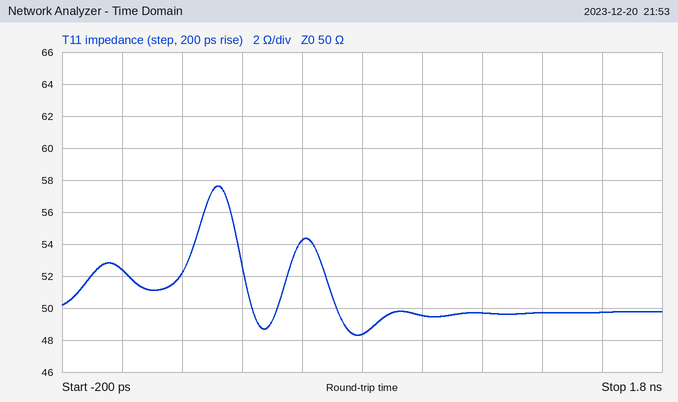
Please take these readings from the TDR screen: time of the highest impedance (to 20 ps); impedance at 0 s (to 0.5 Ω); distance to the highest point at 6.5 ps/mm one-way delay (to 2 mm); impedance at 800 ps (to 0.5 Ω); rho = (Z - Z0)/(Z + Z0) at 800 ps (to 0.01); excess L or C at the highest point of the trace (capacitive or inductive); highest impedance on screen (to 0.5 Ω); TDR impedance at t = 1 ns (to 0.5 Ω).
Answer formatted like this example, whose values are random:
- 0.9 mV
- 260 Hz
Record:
- 320 ps
- 52.5 Ω
- 24 mm
- 48.5 Ω
- -0.02
- inductive
- 57.5 Ω
- 49.5 Ω
